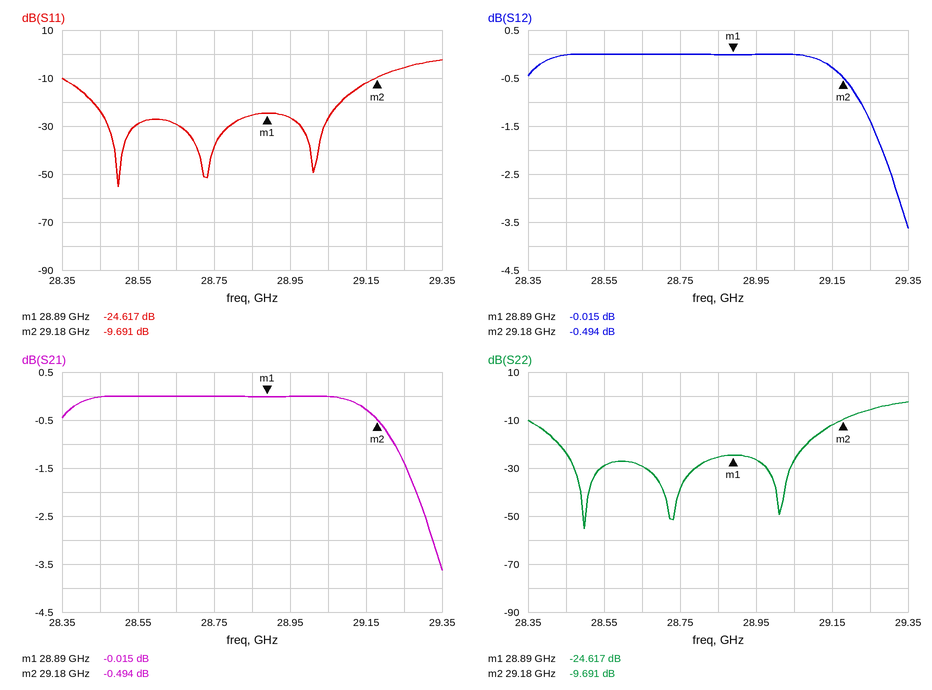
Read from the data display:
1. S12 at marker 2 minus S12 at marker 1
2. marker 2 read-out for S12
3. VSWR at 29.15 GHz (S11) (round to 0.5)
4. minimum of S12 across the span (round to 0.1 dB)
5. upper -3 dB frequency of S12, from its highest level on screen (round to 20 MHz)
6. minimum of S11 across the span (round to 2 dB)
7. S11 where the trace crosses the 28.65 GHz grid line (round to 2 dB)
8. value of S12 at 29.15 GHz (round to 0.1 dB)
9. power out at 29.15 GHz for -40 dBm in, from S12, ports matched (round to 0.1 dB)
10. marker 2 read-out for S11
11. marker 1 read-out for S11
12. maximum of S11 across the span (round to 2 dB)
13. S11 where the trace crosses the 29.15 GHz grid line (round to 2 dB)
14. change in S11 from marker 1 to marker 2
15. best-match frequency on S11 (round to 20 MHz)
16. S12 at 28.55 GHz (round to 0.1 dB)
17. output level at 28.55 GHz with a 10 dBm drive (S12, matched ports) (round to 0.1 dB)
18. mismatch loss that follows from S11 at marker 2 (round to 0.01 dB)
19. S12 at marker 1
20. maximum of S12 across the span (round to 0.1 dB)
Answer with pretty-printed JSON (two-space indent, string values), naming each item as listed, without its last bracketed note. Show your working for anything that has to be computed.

{
  "S12 at marker 2 minus S12 at marker 1": "-0.494 − (-0.015) = -0.479 dB",
  "marker 2 read-out for S12": "-0.494 dB",
  "VSWR at 29.15 GHz (S11)": "|Γ| = 10^(-12/20) = 0.2512; VSWR = (1 + 0.2512)/(1 − 0.2512) ≈ 1.67, so 1.5 to the nearest 0.5",
  "minimum of S12 across the span": "-3.6 dB",
  "upper -3 dB frequency of S12, from its highest level on screen": "29.32 GHz",
  "minimum of S11 across the span": "-56 dB",
  "S11 where the trace crosses the 28.65 GHz grid line": "-30 dB",
  "value of S12 at 29.15 GHz": "-0.3 dB",
  "power out at 29.15 GHz for -40 dBm in, from S12, ports matched": "-40 dBm + (-0.3 dB) = -40.3 dBm",
  "marker 2 read-out for S11": "-9.691 dB",
  "marker 1 read-out for S11": "-24.617 dB",
  "maximum of S11 across the span": "-2 dB",
  "S11 where the trace crosses the 29.15 GHz grid line": "-12 dB",
  "change in S11 from marker 1 to marker 2": "-9.691 − (-24.617) = 14.926 dB",
  "best-match frequency on S11": "28.50 GHz",
  "S12 at 28.55 GHz": "0.0 dB",
  "output level at 28.55 GHz with a 10 dBm drive (S12, matched ports)": "10 dBm + (0.0 dB) = 10.0 dBm",
  "mismatch loss that follows from S11 at marker 2": "−10 log10(1 − 10^(-9.691/10)) ≈ 0.49 dB",
  "S12 at marker 1": "-0.015 dB",
  "maximum of S12 across the span": "0.0 dB"
}
